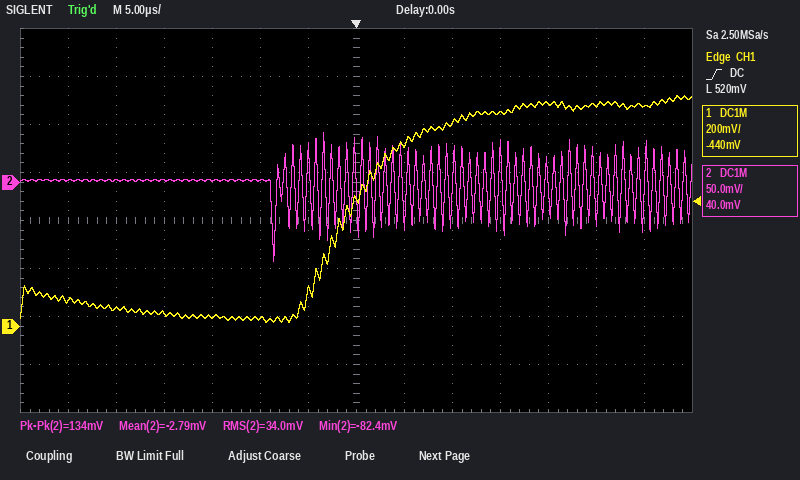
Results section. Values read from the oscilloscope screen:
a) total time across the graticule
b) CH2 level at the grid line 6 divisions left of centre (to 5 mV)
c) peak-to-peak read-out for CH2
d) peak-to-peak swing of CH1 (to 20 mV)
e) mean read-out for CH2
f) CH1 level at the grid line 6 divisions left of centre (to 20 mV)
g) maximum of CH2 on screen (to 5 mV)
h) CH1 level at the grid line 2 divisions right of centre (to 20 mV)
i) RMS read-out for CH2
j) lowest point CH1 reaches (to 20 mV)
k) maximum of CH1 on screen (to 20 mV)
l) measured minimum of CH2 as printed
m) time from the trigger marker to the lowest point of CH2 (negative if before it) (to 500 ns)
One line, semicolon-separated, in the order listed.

70 µs; 0 mV; 134 mV; 940 mV; -2.79 mV; 100 mV; 50 mV; 840 mV; 34.0 mV; 20 mV; 960 mV; -82.4 mV; -8.5 µs
